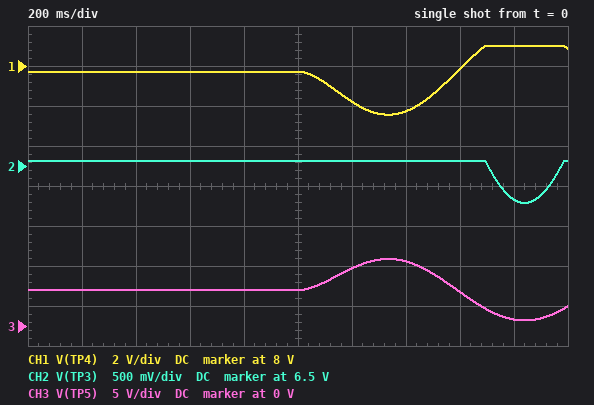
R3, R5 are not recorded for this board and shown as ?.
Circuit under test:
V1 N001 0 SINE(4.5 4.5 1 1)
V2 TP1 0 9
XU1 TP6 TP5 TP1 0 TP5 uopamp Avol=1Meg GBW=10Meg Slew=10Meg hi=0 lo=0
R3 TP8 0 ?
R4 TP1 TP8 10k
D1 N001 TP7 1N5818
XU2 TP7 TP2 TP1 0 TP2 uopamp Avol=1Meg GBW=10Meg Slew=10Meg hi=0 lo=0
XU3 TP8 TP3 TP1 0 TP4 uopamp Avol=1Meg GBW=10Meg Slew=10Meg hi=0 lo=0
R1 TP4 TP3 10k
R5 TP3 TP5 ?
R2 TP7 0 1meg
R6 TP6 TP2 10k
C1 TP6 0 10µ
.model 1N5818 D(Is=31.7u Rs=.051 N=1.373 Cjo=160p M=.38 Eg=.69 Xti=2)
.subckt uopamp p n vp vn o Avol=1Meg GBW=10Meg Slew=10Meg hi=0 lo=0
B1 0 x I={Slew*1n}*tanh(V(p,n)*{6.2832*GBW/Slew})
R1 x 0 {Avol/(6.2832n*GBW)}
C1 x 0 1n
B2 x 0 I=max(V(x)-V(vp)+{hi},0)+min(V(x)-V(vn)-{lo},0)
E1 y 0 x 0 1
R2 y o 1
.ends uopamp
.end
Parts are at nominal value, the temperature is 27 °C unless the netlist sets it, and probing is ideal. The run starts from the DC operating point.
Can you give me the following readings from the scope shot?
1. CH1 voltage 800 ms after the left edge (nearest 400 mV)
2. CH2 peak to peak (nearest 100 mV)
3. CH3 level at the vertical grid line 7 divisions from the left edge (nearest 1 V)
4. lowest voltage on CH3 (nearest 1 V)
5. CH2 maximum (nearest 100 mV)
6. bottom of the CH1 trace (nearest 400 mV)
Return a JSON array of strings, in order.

["7.6 V", "500 mV", "8 V", "1 V", "6.6 V", "5.6 V"]
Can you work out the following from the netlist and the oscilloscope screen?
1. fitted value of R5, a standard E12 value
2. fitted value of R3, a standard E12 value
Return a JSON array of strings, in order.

["18 kΩ", "27 kΩ"]
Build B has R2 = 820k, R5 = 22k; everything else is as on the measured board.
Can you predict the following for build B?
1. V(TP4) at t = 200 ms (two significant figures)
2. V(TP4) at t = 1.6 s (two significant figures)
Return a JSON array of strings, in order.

["7.5 V", "7.6 V"]
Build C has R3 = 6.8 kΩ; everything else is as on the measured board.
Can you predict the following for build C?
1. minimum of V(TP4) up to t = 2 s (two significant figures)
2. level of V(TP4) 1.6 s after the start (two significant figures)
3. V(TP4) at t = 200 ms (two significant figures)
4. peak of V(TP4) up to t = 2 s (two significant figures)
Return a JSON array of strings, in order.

["1.0 V", "3.3 V", "3.2 V", "5.3 V"]
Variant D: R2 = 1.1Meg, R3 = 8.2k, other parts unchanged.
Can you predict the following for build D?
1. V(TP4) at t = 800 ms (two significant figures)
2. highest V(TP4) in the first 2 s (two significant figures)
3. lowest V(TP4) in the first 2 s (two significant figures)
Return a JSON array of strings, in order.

["3.8 V", "5.9 V", "1.7 V"]
